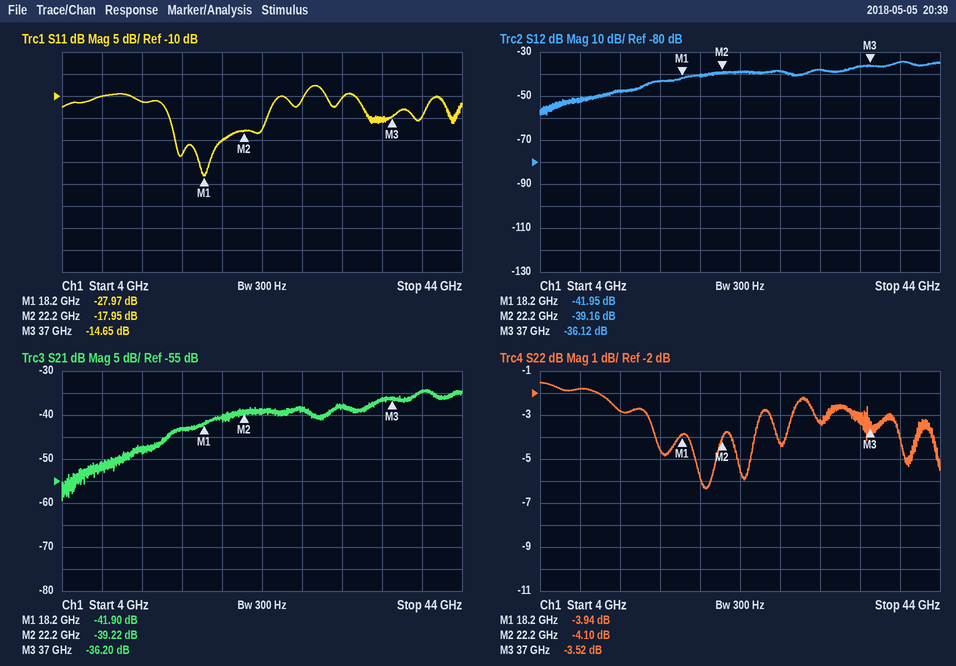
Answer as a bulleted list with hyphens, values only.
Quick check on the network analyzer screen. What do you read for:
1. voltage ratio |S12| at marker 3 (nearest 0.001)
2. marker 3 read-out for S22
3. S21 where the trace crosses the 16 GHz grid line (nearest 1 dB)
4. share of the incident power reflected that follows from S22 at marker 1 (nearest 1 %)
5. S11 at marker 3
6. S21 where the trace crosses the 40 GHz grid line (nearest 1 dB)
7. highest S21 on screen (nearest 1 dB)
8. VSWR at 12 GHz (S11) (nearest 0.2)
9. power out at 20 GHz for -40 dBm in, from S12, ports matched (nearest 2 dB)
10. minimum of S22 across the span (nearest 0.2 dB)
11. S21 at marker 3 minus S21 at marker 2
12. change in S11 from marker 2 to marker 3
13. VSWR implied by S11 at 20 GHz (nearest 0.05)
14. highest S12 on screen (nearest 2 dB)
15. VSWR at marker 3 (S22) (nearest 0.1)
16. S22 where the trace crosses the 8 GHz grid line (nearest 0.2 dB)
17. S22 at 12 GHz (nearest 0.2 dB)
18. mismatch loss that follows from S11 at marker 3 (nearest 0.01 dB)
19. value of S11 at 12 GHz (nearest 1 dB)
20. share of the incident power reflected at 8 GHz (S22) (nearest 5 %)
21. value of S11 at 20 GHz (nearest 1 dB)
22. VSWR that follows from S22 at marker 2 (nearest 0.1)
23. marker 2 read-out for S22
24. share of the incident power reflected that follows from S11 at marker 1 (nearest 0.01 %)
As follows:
- 0.016
- -3.52 dB
- -43 dB
- 40 %
- -14.65 dB
- -35 dB
- -34 dB
- 1.8
- -80 dBm
- -6.4 dB
- 3.02 dB
- 3.30 dB
- 1.20
- -34 dB
- 5.0
- -1.8 dB
- -2.8 dB
- 0.15 dB
- -11 dB
- 65 %
- -20 dB
- 4.3
- -4.10 dB
- 0.16 %
